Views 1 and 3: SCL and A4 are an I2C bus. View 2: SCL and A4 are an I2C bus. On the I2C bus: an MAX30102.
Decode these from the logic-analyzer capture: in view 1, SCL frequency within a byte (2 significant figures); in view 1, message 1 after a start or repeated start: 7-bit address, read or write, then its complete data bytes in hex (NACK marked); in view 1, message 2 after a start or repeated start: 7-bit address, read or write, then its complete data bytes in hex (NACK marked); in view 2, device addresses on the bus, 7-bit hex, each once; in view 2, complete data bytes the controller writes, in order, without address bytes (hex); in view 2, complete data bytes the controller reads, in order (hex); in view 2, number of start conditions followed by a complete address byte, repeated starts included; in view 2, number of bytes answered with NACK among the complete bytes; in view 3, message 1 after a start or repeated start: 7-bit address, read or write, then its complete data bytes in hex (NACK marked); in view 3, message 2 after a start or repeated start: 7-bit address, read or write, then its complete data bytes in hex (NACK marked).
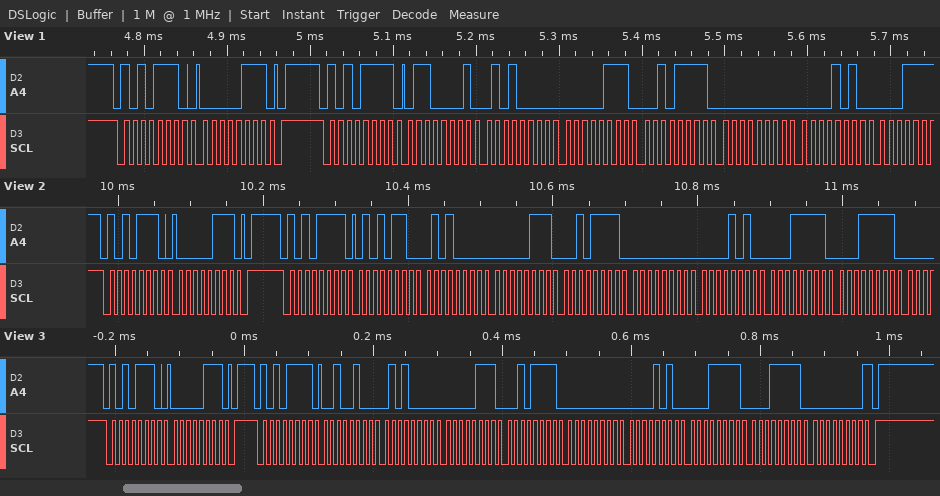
100 kHz
0x57 write: 07
0x57 read: 61 50 07 2F 00 0A
0x57
07
56 50 07 2F 00 0A 1F 1F
2
0
0x57 write: 07
0x57 read: 24 50 07 2F 00 0A 1F 1F 00 NACK
